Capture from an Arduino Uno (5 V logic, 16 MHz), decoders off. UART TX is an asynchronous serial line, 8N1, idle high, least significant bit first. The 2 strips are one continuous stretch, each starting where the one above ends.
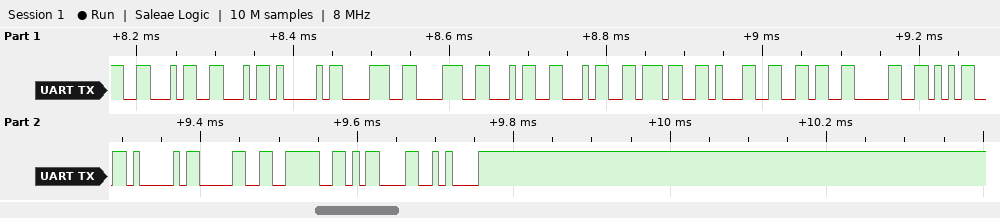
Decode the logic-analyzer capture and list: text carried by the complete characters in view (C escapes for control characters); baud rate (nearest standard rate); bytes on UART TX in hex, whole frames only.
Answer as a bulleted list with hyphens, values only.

- "FFA884471605A0>\r\n"
- 115200 baud
- 46 46 41 38 38 34 34 37 31 36 30 35 41 30 3E 0D 0A
